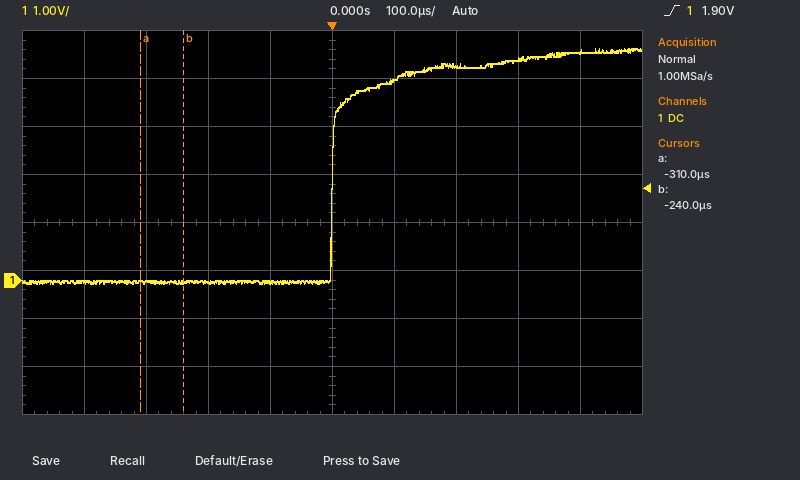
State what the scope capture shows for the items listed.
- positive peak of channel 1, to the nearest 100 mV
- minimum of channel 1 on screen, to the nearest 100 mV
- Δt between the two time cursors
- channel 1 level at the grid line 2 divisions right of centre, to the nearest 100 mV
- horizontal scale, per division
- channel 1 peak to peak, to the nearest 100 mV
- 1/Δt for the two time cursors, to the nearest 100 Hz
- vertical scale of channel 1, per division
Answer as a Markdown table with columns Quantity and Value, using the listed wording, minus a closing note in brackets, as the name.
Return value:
| Quantity | Value |
|---|---|
| positive peak of channel 1, to the nearest 100 mV | 4.8 V |
| minimum of channel 1 on screen, to the nearest 100 mV | -100 mV |
| Δt between the two time cursors | 70 µs |
| channel 1 level at the grid line 2 divisions right of centre, to the nearest 100 mV | 4.5 V |
| horizontal scale, per division | 100 µs |
| channel 1 peak to peak, to the nearest 100 mV | 4.9 V |
| 1/Δt for the two time cursors, to the nearest 100 Hz | 14.3 kHz |
| vertical scale of channel 1, per division | 1 V |
